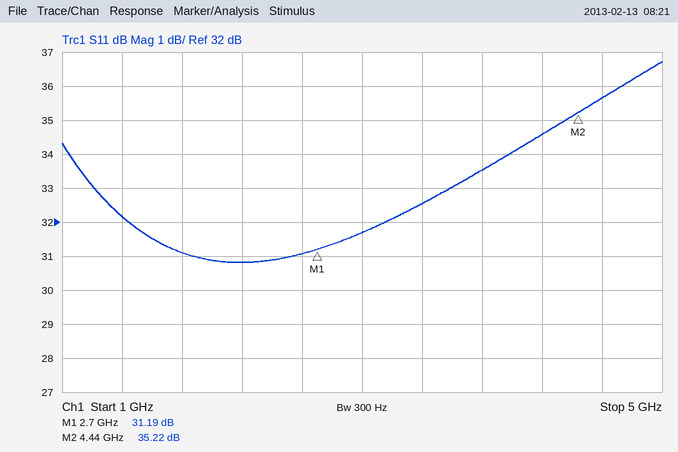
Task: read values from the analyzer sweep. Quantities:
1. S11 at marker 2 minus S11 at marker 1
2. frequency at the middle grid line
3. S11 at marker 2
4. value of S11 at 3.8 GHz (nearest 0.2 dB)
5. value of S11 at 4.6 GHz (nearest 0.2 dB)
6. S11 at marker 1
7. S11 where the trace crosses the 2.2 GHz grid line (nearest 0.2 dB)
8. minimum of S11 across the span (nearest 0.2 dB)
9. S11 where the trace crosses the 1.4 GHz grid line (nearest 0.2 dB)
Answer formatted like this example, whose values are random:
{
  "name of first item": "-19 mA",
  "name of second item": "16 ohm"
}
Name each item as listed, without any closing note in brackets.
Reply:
{
  "S11 at marker 2 minus S11 at marker 1": "4.03 dB",
  "frequency at the middle grid line": "3 GHz",
  "S11 at marker 2": "35.22 dB",
  "value of S11 at 3.8 GHz": "33.6 dB",
  "value of S11 at 4.6 GHz": "35.6 dB",
  "S11 at marker 1": "31.19 dB",
  "S11 where the trace crosses the 2.2 GHz grid line": "30.8 dB",
  "minimum of S11 across the span": "30.8 dB",
  "S11 where the trace crosses the 1.4 GHz grid line": "32.2 dB"
}
